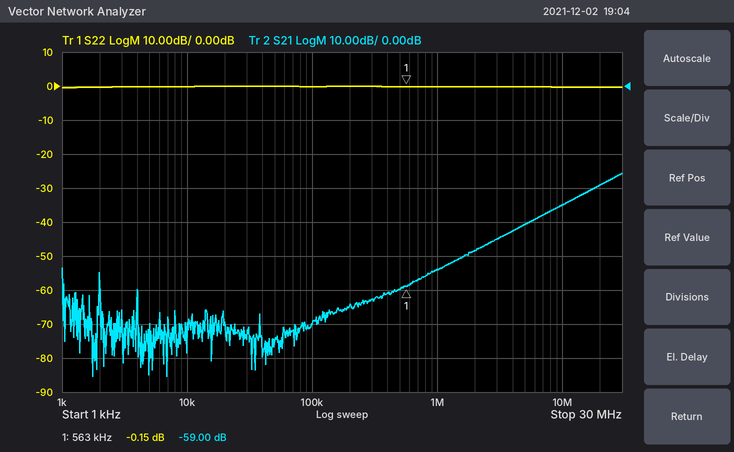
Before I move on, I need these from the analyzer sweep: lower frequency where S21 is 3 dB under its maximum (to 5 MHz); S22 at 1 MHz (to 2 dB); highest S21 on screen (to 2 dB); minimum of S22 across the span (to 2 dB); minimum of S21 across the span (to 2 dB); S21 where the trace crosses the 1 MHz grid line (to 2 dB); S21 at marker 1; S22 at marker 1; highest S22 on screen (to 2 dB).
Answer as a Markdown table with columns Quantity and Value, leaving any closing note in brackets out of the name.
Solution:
| Quantity | Value |
|---|---|
| lower frequency where S21 is 3 dB under its maximum | 20 MHz |
| S22 at 1 MHz | 0 dB |
| highest S21 on screen | -26 dB |
| minimum of S22 across the span | 0 dB |
| minimum of S21 across the span | -86 dB |
| S21 where the trace crosses the 1 MHz grid line | -54 dB |
| S21 at marker 1 | -59.00 dB |
| S22 at marker 1 | -0.15 dB |
| highest S22 on screen | 0 dB |
